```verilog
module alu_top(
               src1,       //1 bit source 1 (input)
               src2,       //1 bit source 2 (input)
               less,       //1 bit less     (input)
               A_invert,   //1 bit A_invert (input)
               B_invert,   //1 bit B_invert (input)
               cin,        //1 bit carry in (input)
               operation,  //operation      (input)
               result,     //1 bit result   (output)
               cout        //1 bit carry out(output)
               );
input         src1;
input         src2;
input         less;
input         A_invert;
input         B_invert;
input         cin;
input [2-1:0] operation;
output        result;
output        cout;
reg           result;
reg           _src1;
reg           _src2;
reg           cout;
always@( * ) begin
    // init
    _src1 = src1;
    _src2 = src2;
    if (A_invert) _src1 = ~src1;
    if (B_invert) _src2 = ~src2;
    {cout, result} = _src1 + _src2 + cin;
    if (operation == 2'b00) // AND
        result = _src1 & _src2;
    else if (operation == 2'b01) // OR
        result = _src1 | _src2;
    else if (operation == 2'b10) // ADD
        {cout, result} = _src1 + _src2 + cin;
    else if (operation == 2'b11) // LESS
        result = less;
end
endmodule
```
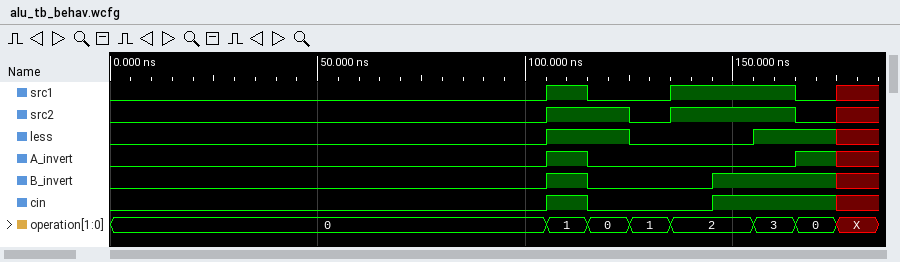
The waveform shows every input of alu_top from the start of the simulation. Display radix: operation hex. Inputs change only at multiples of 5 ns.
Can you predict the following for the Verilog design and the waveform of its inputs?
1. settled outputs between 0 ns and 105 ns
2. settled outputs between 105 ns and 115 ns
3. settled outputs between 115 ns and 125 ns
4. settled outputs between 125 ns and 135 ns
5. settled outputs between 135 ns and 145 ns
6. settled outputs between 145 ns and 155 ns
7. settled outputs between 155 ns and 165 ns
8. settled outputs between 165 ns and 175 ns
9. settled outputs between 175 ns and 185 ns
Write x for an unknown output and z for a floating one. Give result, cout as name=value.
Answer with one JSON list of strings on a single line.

["result=0, cout=0", "result=0, cout=0", "result=0, cout=0", "result=0, cout=0", "result=0, cout=1", "result=0, cout=1", "result=1, cout=1", "result=1, cout=1", "result=x, cout=x"]
